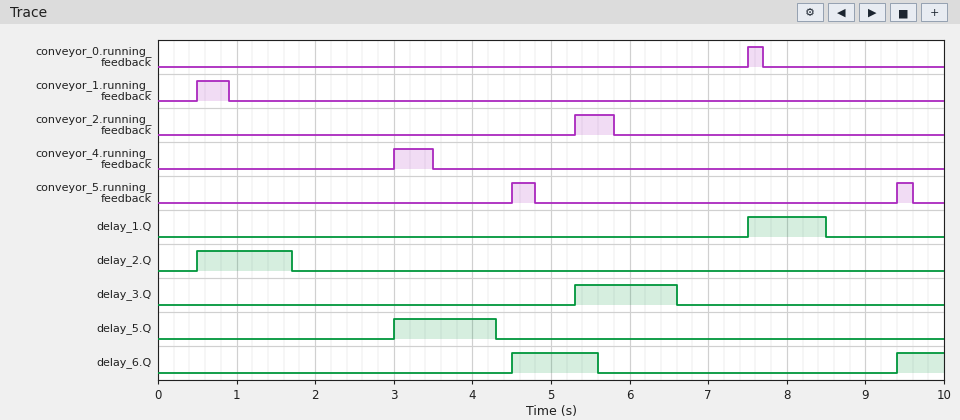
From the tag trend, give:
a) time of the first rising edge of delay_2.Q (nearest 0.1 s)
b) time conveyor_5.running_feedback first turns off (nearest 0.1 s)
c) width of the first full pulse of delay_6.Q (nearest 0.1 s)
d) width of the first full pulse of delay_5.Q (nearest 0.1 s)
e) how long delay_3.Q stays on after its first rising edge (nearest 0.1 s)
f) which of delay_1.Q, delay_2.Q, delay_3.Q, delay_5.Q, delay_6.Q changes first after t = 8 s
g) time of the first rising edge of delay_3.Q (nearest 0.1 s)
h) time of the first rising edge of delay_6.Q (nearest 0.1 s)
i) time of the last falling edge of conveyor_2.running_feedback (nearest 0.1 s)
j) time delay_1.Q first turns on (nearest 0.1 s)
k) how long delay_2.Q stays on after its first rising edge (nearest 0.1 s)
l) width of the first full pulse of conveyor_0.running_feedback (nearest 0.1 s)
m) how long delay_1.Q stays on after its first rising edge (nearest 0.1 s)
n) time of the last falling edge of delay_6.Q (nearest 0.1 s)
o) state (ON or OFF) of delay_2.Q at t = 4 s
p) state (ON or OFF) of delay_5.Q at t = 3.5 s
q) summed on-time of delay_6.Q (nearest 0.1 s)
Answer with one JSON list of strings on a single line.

["0.5 s", "4.8 s", "1.1 s", "1.3 s", "1.3 s", "delay_1.Q", "5.3 s", "4.5 s", "5.8 s", "7.5 s", "1.2 s", "0.2 s", "1.0 s", "5.6 s", "OFF", "ON", "1.7 s"]
